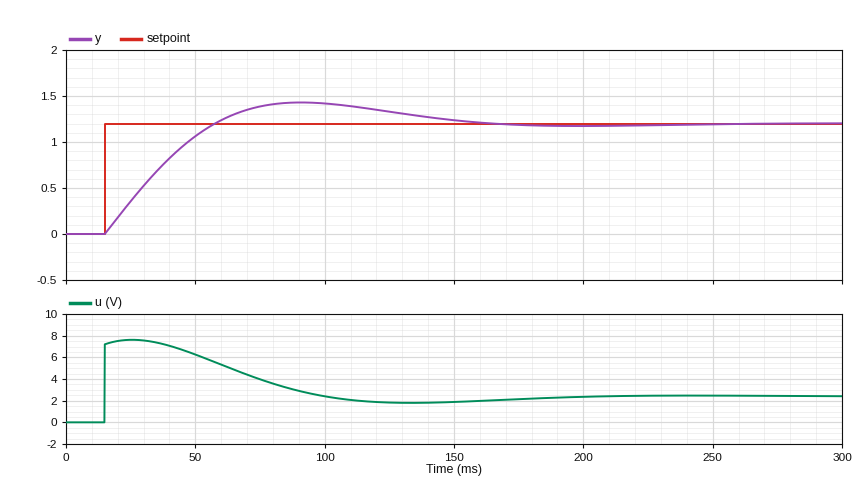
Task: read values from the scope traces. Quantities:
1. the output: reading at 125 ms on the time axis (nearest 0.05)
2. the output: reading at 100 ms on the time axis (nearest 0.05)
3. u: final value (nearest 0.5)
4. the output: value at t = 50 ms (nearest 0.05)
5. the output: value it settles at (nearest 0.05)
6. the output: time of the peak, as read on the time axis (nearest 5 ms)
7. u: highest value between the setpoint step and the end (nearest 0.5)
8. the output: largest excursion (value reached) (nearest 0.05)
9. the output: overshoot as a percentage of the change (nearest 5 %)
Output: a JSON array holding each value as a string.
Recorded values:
["1.35", "1.40", "2.5", "1.05", "1.20", "90 ms", "7.5", "1.45", "20 %"]
